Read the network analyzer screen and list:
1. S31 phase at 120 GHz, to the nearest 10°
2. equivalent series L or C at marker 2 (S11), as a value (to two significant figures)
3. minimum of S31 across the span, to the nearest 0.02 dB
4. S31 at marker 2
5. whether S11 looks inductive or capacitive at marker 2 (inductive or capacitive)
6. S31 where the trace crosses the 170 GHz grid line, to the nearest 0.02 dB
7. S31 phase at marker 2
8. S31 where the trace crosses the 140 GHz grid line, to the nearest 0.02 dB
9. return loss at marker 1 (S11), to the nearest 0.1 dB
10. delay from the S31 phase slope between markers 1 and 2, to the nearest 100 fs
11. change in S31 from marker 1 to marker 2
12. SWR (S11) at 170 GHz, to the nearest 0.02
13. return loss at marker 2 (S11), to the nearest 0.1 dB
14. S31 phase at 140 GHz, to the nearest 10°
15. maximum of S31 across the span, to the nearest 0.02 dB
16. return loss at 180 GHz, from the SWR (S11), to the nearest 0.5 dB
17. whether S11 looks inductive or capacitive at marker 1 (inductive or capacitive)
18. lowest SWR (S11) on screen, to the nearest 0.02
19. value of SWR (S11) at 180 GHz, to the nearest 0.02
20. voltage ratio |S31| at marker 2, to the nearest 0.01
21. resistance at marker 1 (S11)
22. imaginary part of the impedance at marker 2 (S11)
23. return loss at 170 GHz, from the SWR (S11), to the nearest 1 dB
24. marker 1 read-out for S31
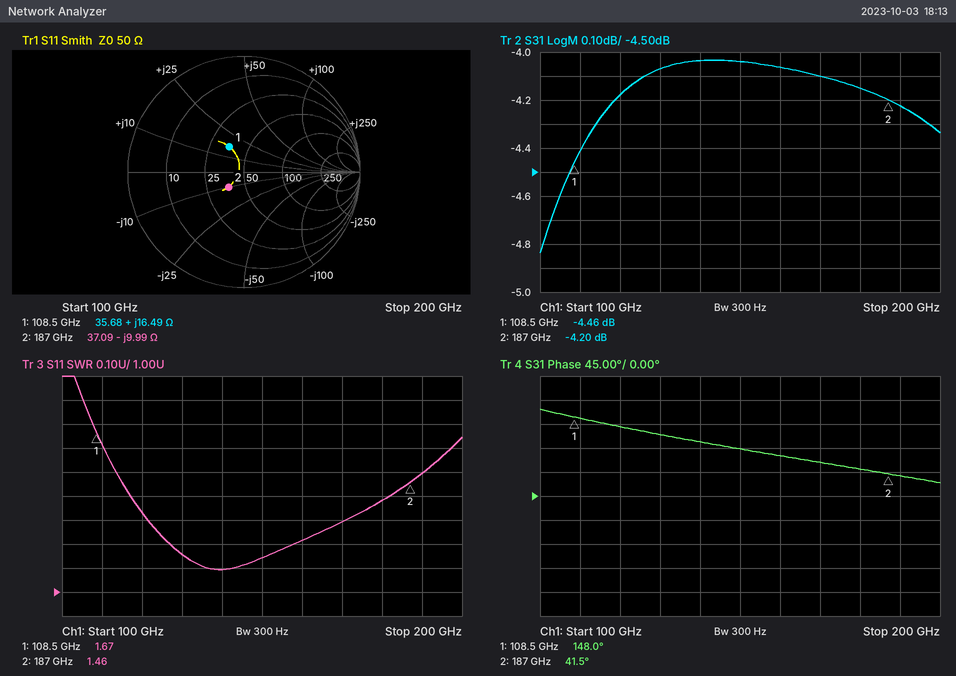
130°
85 fF
-4.84 dB
-4.20 dB
capacitive
-4.10 dB
41.5°
-4.04 dB
12.0 dB
3.8 ps
0.26 dB
1.30
14.6 dB
100°
-4.04 dB
16.0 dB
inductive
1.10
1.38
0.62
35.68 Ω
-9.99 Ω
18 dB
-4.46 dB
